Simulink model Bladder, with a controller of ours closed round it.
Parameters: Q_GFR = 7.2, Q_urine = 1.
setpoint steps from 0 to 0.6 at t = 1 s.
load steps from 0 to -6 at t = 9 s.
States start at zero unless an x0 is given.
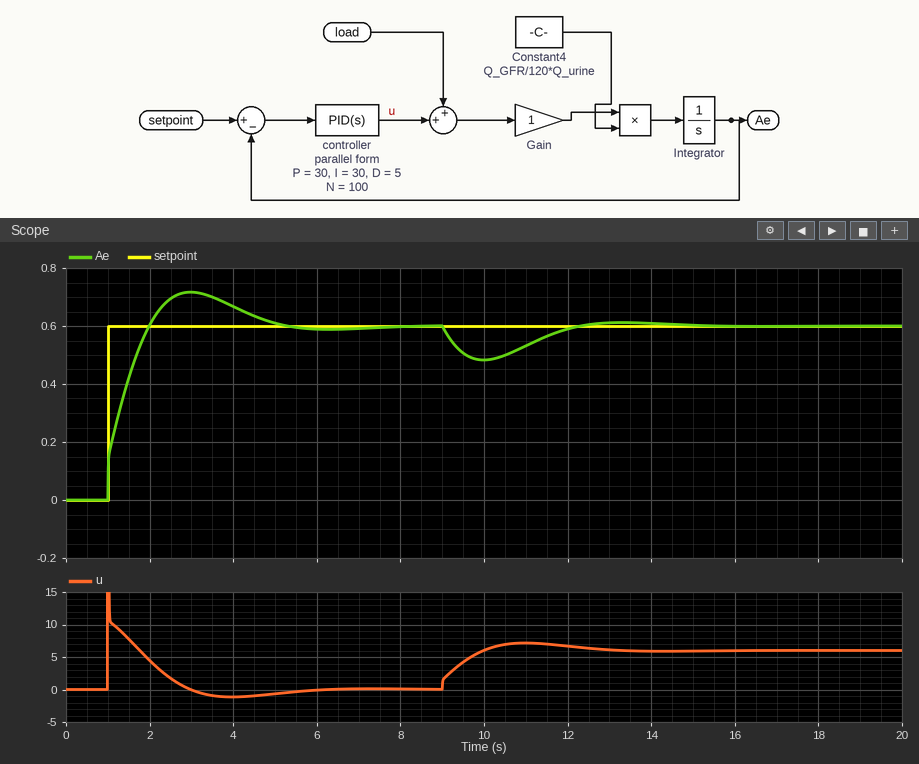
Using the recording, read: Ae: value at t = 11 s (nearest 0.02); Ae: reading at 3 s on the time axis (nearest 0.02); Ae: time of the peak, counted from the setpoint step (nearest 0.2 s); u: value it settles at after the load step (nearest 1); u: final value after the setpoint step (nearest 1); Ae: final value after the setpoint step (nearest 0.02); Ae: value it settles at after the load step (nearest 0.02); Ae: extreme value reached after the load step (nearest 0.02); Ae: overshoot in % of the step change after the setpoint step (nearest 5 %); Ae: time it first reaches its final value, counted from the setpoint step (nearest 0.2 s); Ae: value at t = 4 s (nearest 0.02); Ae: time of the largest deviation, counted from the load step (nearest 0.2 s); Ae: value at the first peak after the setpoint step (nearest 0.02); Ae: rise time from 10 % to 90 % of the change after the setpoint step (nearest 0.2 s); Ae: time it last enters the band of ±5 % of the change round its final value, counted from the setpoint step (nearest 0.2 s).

0.54
0.72
2.0 s
6
0
0.60
0.60
0.48
20 %
1.0 s
0.66
1.0 s
0.72
0.8 s
3.6 s
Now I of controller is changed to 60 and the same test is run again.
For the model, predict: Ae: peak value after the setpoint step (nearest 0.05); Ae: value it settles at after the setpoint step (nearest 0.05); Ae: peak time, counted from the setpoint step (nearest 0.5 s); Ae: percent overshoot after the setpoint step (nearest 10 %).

0.75
0.60
1.5 s
30 %
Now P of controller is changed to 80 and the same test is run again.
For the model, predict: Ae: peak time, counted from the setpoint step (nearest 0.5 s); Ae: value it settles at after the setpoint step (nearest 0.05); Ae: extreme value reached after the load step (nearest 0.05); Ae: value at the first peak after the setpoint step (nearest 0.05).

1.5 s
0.60
0.55
0.65
